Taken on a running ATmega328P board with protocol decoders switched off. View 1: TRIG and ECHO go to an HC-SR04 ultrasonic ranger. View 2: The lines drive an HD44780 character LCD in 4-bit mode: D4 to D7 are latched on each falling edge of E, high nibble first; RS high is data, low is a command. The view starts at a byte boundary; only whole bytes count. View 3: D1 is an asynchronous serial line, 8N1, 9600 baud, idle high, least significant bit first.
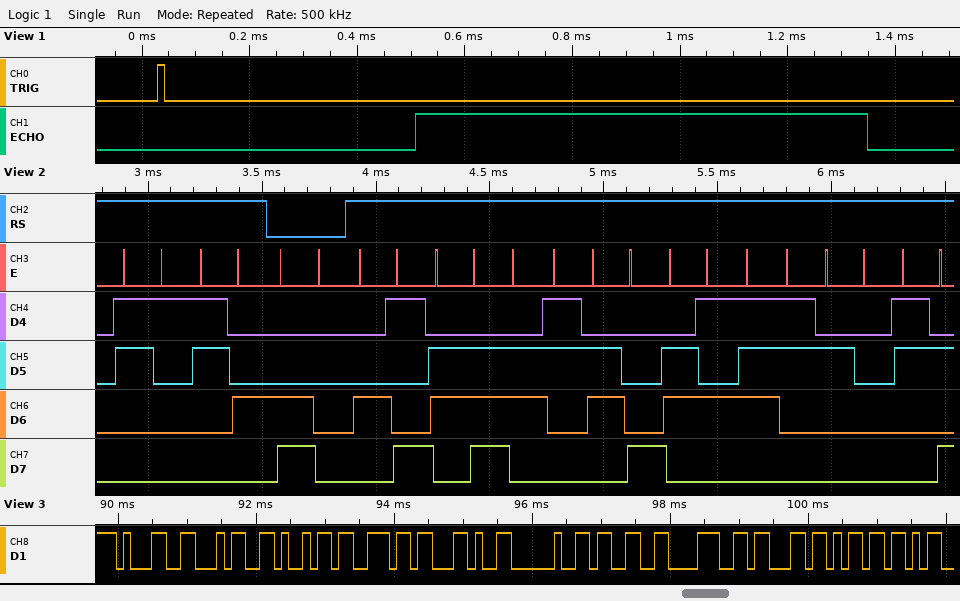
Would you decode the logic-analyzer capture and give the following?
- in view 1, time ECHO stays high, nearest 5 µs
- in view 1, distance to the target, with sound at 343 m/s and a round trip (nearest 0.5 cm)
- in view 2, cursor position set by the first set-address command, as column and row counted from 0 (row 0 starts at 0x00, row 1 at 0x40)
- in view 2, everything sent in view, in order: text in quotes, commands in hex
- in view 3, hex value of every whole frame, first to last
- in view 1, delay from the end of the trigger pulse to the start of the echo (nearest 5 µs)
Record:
840 µs
14.5 cm
column 0, row 1
"14" 0xC0 "Inches :"
31 34 69 6E 2C 20 33 38 63 6D
465 µs
